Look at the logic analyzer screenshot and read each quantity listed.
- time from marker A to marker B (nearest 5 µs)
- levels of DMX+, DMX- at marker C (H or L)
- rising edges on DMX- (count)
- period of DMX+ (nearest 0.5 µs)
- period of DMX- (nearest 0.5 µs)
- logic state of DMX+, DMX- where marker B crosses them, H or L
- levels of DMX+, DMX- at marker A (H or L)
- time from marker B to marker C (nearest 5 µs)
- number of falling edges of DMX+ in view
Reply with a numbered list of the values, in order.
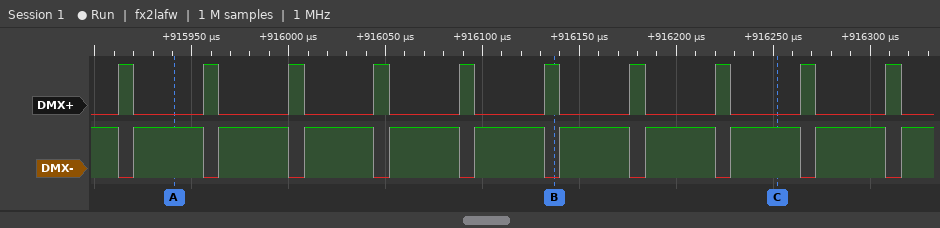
1. 195 µs
2. DMX+=L, DMX-=H
3. 10
4. 44 µs
5. 44 µs
6. DMX+=H, DMX-=L
7. DMX+=L, DMX-=H
8. 115 µs
9. 10
